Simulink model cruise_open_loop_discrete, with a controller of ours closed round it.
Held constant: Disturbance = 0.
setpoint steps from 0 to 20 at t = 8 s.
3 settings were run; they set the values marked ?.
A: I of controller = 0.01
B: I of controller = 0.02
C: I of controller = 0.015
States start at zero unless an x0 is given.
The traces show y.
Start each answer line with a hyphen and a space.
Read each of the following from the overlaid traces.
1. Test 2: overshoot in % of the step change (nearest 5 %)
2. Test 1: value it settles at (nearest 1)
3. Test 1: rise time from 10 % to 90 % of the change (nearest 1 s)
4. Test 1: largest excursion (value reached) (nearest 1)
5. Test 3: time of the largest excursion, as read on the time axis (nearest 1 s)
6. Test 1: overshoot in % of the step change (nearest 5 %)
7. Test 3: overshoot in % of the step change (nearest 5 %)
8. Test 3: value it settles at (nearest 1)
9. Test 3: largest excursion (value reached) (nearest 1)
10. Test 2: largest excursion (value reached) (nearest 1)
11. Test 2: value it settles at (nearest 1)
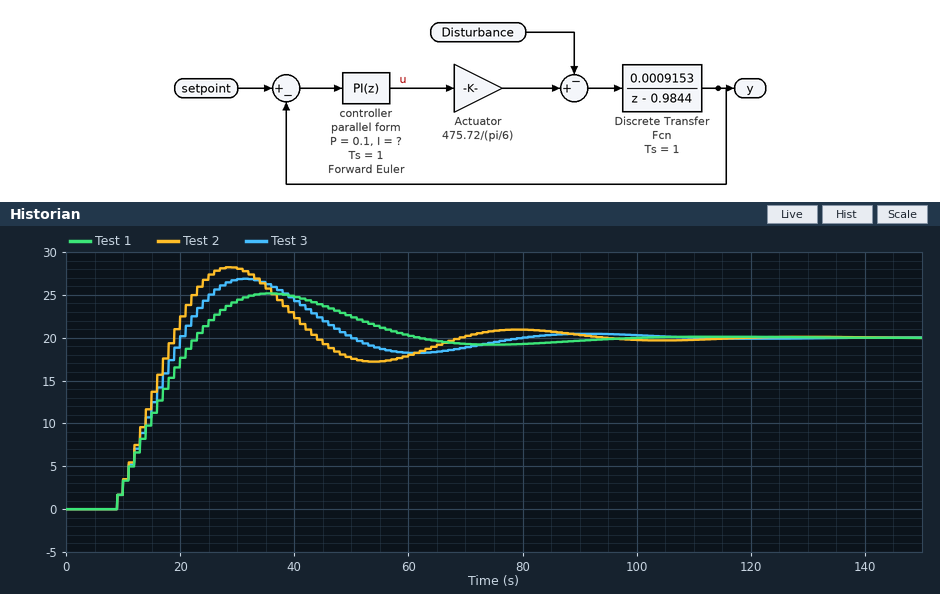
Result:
- 40 %
- 20
- 11 s
- 25
- 31 s
- 25 %
- 35 %
- 20
- 27
- 28
- 20
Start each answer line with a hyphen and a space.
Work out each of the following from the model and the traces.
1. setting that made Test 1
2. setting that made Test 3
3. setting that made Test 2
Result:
- A
- C
- B
